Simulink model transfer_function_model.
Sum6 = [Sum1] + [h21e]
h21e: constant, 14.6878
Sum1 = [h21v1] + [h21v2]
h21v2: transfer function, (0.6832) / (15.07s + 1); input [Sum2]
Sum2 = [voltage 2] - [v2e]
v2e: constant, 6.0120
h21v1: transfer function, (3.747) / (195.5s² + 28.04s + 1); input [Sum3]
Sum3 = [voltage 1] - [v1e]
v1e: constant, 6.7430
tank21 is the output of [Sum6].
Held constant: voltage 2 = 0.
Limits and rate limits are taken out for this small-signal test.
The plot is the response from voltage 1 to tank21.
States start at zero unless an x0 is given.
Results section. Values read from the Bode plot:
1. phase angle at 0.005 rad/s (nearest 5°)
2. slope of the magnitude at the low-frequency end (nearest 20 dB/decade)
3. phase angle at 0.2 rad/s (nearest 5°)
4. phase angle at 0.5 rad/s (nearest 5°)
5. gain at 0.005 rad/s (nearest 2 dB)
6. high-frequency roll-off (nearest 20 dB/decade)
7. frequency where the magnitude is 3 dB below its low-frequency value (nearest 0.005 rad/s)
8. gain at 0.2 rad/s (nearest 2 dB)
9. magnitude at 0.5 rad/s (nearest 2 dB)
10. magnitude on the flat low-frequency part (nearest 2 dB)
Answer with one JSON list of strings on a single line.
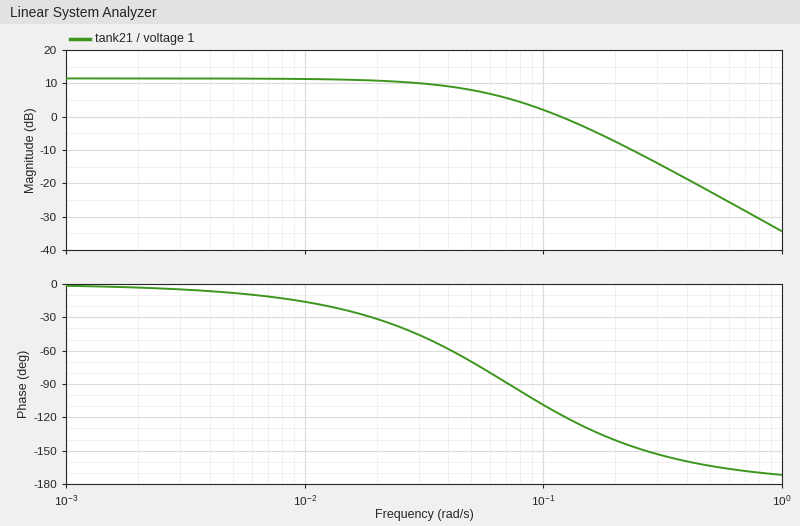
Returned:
["-10°", "0 dB/decade", "-140°", "-165°", "12 dB", "-40 dB/decade", "0.045 rad/s", "-8 dB", "-22 dB", "12 dB"]
